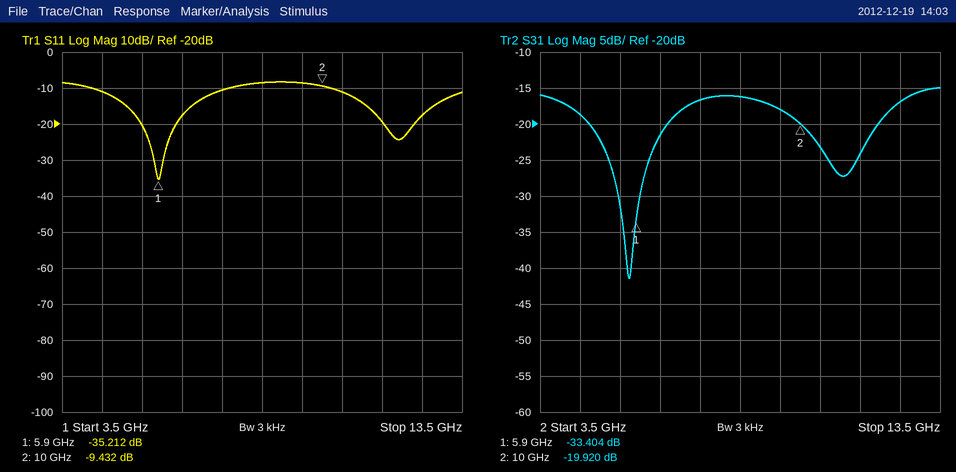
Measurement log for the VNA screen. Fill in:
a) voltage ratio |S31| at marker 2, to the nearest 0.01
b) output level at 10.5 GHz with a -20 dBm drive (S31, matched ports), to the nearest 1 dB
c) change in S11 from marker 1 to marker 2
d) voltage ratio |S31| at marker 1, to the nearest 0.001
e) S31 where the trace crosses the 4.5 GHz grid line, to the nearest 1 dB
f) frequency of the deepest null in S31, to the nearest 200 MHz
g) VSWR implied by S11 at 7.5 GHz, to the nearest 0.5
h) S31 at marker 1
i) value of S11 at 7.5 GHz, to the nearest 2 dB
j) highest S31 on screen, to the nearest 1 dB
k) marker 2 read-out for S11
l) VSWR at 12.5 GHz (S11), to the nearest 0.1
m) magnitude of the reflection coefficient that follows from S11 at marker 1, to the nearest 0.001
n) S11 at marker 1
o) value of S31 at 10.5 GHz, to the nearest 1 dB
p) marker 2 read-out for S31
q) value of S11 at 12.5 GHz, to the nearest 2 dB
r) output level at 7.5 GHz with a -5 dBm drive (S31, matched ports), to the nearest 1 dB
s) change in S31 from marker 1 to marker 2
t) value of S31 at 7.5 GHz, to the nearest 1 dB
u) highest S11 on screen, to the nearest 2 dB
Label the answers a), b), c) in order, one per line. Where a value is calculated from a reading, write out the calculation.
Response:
a) 10^(-19.92/20) ≈ 0.10
b) -20 dBm + (-23 dB) = -43 dBm
c) -9.432 − (-35.212) = 25.780 dB
d) 10^(-33.404/20) ≈ 0.021
e) -19 dB
f) 5.8 GHz
g) |Γ| = 10^(-10/20) = 0.3162; VSWR = (1 + 0.3162)/(1 − 0.3162) ≈ 1.92, so 2.0 to the nearest 0.5
h) -33.404 dB
i) -10 dB
j) -15 dB
k) -9.432 dB
l) |Γ| = 10^(-18/20) = 0.1259; VSWR = (1 + 0.1259)/(1 − 0.1259) ≈ 1.3
m) 10^(-35.212/20) ≈ 0.017
n) -35.212 dB
o) -23 dB
p) -19.920 dB
q) -18 dB
r) -5 dBm + (-17 dB) = -22 dBm
s) -19.92 − (-33.404) = 13.484 dB
t) -17 dB
u) -8 dB
